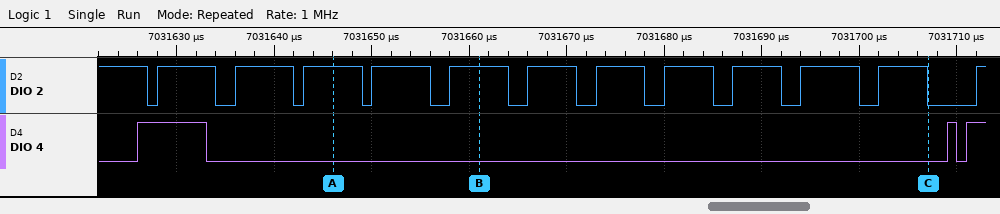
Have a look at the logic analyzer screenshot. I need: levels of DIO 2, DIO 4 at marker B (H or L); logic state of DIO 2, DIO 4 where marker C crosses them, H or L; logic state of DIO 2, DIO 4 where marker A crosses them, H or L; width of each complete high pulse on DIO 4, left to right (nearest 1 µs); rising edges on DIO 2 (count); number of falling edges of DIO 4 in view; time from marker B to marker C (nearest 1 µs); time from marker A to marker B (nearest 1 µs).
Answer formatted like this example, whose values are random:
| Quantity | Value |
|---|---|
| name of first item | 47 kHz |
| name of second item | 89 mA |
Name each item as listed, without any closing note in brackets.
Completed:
| Quantity | Value |
|---|---|
| levels of DIO 2, DIO 4 at marker B | DIO 2=H, DIO 4=L |
| logic state of DIO 2, DIO 4 where marker C crosses them, H or L | DIO 2=L, DIO 4=L |
| logic state of DIO 2, DIO 4 where marker A crosses them, H or L | DIO 2=H, DIO 4=L |
| width of each complete high pulse on DIO 4, left to right | 7 µs, 1 µs |
| rising edges on DIO 2 | 12 |
| number of falling edges of DIO 4 in view | 2 |
| time from marker B to marker C | 46 µs |
| time from marker A to marker B | 15 µs |
